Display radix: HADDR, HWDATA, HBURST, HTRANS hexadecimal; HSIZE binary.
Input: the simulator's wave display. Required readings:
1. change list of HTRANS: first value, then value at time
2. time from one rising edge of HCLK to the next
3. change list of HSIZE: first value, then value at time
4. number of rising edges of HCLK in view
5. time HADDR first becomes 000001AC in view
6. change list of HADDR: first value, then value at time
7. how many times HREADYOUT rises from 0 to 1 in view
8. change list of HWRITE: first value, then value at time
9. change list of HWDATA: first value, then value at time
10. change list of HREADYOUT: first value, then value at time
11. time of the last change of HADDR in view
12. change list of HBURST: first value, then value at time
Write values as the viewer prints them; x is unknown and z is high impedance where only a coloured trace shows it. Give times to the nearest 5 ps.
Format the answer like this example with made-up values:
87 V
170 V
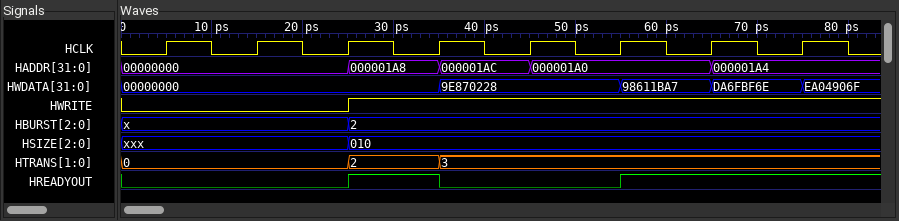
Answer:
0, 2 at 25 ps, 3 at 35 ps
10 ps
xxx, 010 at 25 ps
8
35 ps
00000000, 000001A8 at 25 ps, 000001AC at 35 ps, 000001A0 at 45 ps, 000001A4 at 65 ps
2
0, 1 at 25 ps
00000000, 9E870228 at 35 ps, 98611BA7 at 55 ps, DA6FBF6E at 65 ps, EA04906F at 75 ps
0, 1 at 25 ps, 0 at 35 ps, 1 at 55 ps
65 ps
x, 2 at 25 ps
